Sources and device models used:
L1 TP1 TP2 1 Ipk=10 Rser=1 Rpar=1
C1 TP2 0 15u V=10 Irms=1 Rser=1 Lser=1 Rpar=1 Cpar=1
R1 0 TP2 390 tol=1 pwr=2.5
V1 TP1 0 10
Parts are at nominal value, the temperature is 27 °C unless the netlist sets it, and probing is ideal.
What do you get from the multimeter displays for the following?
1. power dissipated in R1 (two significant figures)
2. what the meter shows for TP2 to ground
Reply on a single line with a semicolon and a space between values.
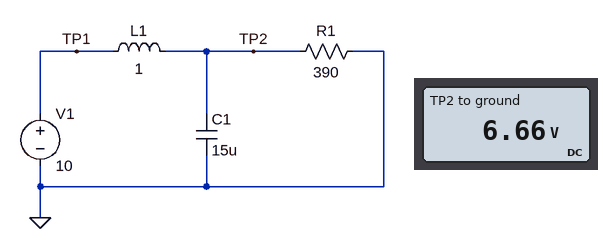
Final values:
110 mW; 6.66 V
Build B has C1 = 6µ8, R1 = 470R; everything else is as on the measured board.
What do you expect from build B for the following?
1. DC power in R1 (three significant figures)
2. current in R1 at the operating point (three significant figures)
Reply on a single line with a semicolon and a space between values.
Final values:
94.4 mW; 14.2 mA
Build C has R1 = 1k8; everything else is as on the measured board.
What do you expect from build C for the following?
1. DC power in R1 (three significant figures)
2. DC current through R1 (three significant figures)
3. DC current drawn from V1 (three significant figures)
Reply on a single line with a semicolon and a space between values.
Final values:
24.7 mW; 3.70 mA; 6.67 A
